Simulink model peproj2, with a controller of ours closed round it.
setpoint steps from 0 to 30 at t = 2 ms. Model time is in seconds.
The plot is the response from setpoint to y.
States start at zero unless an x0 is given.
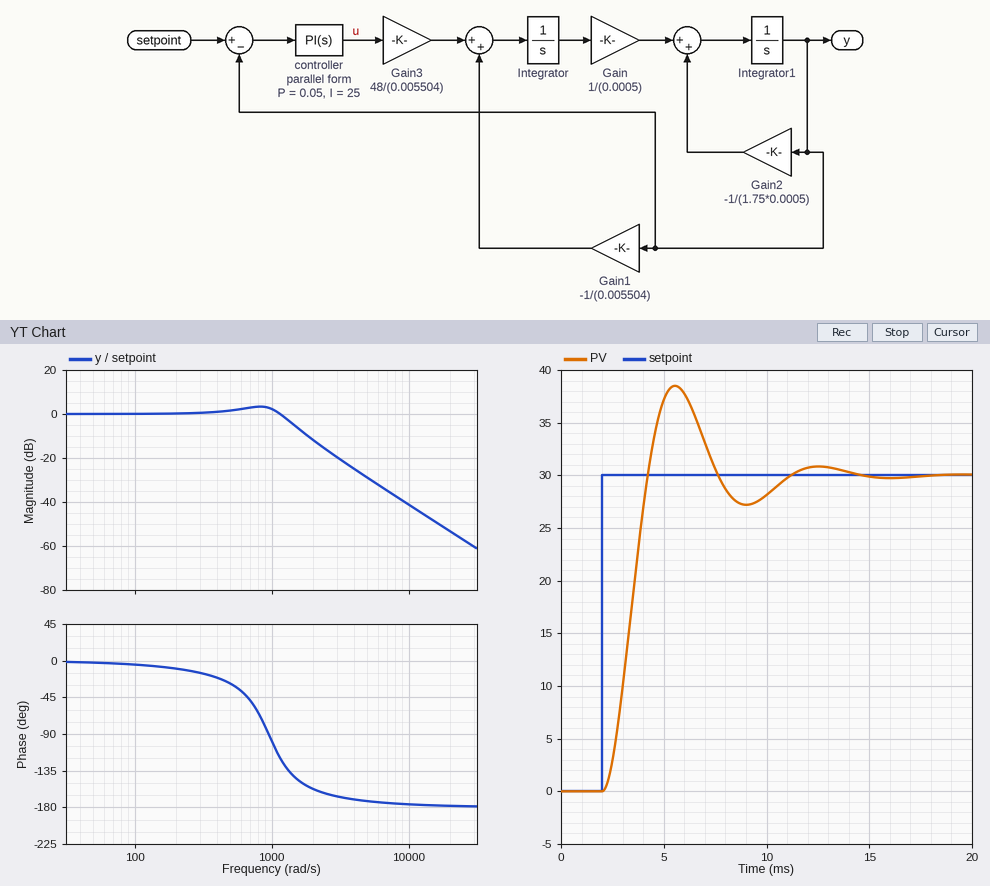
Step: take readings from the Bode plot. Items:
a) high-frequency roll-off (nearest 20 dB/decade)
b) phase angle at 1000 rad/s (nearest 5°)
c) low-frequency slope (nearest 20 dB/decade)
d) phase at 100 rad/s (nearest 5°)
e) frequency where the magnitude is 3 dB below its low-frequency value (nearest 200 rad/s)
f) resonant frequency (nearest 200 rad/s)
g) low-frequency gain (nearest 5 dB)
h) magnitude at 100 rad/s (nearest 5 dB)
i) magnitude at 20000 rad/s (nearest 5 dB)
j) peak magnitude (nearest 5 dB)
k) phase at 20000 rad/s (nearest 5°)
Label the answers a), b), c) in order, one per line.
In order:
a) -40 dB/decade
b) -100°
c) 0 dB/decade
d) -5°
e) 1400 rad/s
f) 800 rad/s
g) 0 dB
h) 0 dB
i) -55 dB
j) 5 dB
k) -180°
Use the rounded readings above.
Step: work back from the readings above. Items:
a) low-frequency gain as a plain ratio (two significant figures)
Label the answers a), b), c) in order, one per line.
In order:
a) 1.0
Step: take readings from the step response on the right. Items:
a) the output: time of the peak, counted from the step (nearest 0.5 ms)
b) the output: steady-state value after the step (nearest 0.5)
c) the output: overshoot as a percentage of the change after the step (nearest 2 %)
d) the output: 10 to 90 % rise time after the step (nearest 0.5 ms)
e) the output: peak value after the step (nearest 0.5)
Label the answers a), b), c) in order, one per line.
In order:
a) 3.5 ms
b) 30.0
c) 28 %
d) 1.5 ms
e) 38.5
